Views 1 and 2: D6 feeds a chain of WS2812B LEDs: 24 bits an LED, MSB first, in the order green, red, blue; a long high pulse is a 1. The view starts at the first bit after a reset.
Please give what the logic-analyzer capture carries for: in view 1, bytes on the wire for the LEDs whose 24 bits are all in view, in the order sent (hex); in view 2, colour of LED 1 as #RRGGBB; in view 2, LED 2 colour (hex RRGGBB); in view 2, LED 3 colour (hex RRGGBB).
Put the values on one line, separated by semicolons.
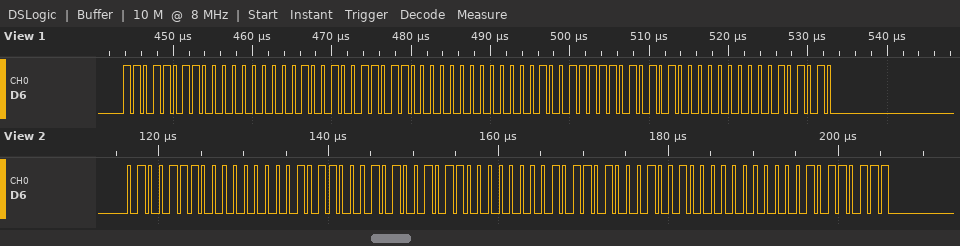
DB 00 24 D8 00 27 D5 00 2A; #004EB1; #004BB4; #0048B7
